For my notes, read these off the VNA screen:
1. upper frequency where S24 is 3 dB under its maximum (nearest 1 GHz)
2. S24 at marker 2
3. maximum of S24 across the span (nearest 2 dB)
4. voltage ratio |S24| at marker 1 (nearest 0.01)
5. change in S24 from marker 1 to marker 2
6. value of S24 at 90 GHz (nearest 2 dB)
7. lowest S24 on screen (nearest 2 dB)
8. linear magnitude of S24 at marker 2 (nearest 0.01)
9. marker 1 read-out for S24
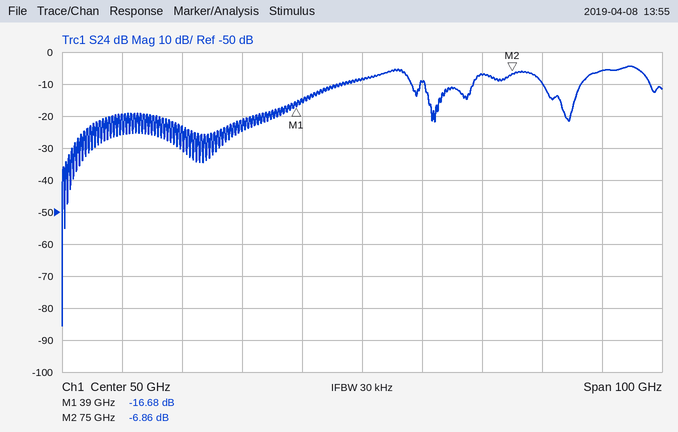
97 GHz
-6.86 dB
-4 dB
0.15
9.82 dB
-6 dB
-86 dB
0.45
-16.68 dB
